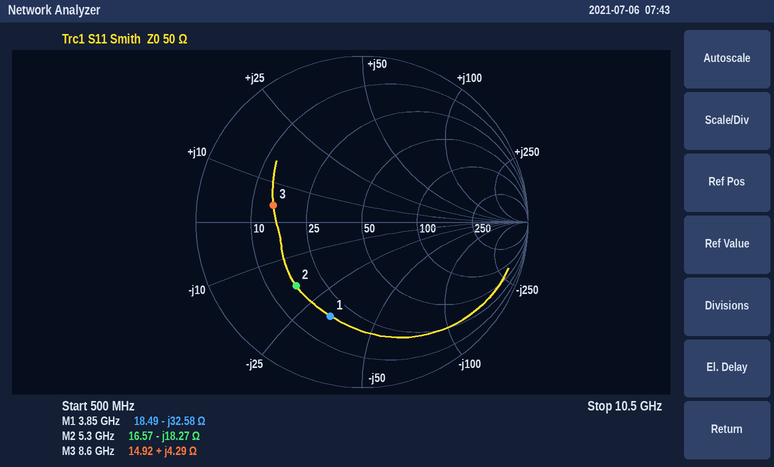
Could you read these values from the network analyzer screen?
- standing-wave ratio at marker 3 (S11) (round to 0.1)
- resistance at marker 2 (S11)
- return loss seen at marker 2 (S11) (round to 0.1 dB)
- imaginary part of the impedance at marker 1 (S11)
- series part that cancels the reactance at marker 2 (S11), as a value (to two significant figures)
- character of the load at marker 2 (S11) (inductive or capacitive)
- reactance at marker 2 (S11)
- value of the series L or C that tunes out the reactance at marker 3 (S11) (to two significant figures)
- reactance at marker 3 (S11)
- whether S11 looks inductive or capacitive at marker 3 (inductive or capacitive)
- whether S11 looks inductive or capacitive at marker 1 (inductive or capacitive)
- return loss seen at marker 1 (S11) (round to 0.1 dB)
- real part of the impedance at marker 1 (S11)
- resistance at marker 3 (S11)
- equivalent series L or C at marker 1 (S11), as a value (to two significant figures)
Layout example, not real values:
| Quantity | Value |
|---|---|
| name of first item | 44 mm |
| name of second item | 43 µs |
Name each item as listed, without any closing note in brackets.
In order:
| Quantity | Value |
|---|---|
| standing-wave ratio at marker 3 (S11) | 3.4 |
| resistance at marker 2 | 16.57 Ω |
| return loss seen at marker 2 (S11) | 5.2 dB |
| imaginary part of the impedance at marker 1 | -32.58 Ω |
| series part that cancels the reactance at marker 2 (S11), as a value | 550 pH |
| character of the load at marker 2 (S11) | capacitive |
| reactance at marker 2 | -18.27 Ω |
| value of the series L or C that tunes out the reactance at marker 3 (S11) | 4.3 pF |
| reactance at marker 3 | +4.29 Ω |
| whether S11 looks inductive or capacitive at marker 3 | inductive |
| whether S11 looks inductive or capacitive at marker 1 | capacitive |
| return loss seen at marker 1 (S11) | 4.5 dB |
| real part of the impedance at marker 1 | 18.49 Ω |
| resistance at marker 3 | 14.92 Ω |
| equivalent series L or C at marker 1 (S11), as a value | 1.3 pF |
